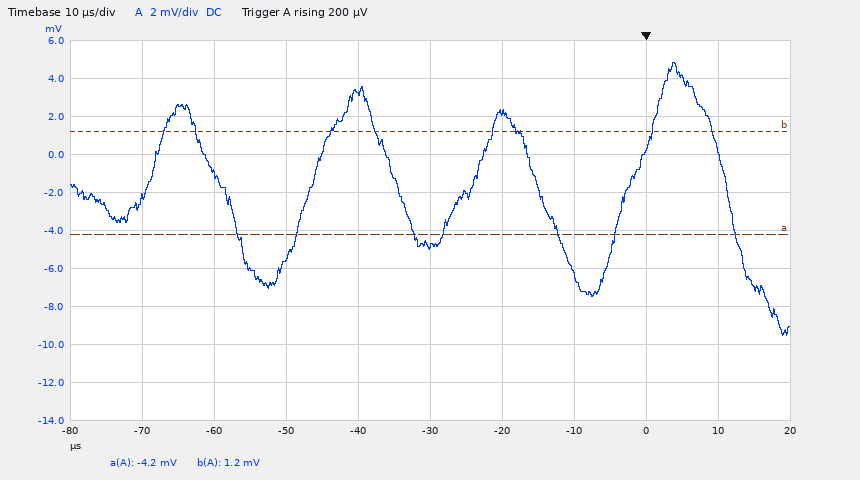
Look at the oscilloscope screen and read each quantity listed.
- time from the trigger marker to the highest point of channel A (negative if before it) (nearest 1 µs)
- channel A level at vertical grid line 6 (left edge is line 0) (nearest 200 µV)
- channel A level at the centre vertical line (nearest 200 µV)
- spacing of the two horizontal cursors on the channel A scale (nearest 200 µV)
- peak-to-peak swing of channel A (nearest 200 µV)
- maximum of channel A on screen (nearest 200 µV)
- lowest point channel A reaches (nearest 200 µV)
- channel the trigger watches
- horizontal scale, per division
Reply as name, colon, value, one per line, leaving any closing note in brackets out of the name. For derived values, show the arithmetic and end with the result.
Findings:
time from the trigger marker to the highest point of channel A (negative if before it): +4 µs
channel A level at vertical grid line 6 (left edge is line 0): 2.2 mV
channel A level at the centre vertical line: -4.8 mV
spacing of the two horizontal cursors on the channel A scale: 5.4 mV
peak-to-peak swing of channel A: 4.8 mV − (-9.6 mV) = 14.4 mV
maximum of channel A on screen: 4.8 mV
lowest point channel A reaches: -9.6 mV
channel the trigger watches: channel A
horizontal scale, per division: 10 µs
